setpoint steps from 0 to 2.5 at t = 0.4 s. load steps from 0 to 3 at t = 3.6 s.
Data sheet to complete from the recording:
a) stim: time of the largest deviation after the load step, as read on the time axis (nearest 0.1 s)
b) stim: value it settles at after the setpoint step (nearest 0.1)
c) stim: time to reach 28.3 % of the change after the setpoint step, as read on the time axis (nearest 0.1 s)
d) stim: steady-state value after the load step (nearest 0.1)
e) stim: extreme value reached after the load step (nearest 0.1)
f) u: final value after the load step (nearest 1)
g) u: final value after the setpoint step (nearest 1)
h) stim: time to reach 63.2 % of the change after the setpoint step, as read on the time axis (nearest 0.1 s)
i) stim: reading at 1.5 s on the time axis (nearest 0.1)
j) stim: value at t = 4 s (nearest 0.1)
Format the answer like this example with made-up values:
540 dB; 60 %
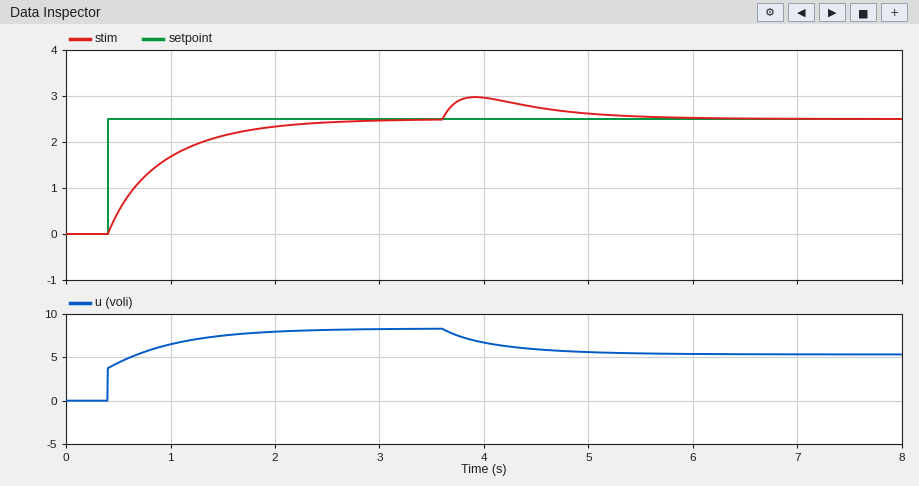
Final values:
3.9 s; 2.5; 0.6 s; 2.5; 3.0; 5; 8; 0.9 s; 2.1; 3.0
